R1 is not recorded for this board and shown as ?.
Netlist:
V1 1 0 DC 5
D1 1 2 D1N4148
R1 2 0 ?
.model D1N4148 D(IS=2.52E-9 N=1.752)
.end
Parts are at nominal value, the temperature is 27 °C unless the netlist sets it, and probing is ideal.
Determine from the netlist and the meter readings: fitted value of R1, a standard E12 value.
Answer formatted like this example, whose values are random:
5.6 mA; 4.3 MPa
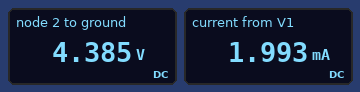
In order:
2.2 kΩ
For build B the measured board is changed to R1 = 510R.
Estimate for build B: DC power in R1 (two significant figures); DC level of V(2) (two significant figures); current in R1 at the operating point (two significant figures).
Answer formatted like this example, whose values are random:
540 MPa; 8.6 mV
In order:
37 mW; 4.3 V; 8.5 mA
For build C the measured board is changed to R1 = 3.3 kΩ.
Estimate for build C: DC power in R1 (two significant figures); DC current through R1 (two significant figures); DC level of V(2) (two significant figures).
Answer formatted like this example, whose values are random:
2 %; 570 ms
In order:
5.9 mW; 1.3 mA; 4.4 V
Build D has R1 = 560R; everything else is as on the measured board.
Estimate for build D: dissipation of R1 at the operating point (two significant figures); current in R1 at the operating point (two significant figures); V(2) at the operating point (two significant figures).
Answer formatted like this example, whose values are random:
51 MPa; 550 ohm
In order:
33 mW; 7.7 mA; 4.3 V
